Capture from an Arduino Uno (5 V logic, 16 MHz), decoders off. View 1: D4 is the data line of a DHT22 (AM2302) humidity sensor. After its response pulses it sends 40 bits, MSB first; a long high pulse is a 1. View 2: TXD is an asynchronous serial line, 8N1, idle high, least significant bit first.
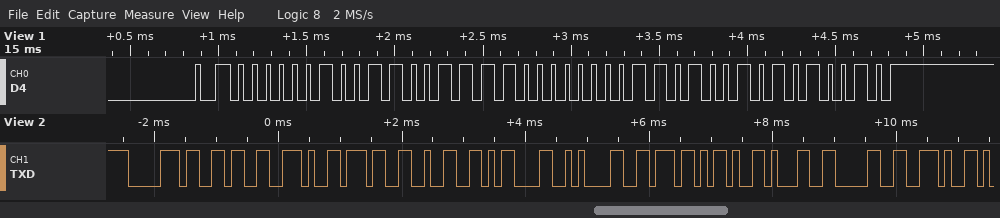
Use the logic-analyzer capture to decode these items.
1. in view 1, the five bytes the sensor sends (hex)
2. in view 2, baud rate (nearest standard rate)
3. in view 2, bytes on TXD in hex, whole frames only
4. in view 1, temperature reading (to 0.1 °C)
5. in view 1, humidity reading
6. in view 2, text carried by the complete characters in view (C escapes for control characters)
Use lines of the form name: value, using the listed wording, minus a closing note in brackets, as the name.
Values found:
in view 1, the five bytes the sensor sends: 02 67 80 69 52
in view 2, baud rate: 9600 baud
in view 2, bytes on TXD in hex, whole frames only: 70 36 2E 37 32 0D 0A 76 2D 31 30 2E
in view 1, temperature reading: -10.5 °C
in view 1, humidity reading: 61.5 %
in view 2, text carried by the complete characters in view: "p6.72\r\nv-10."
